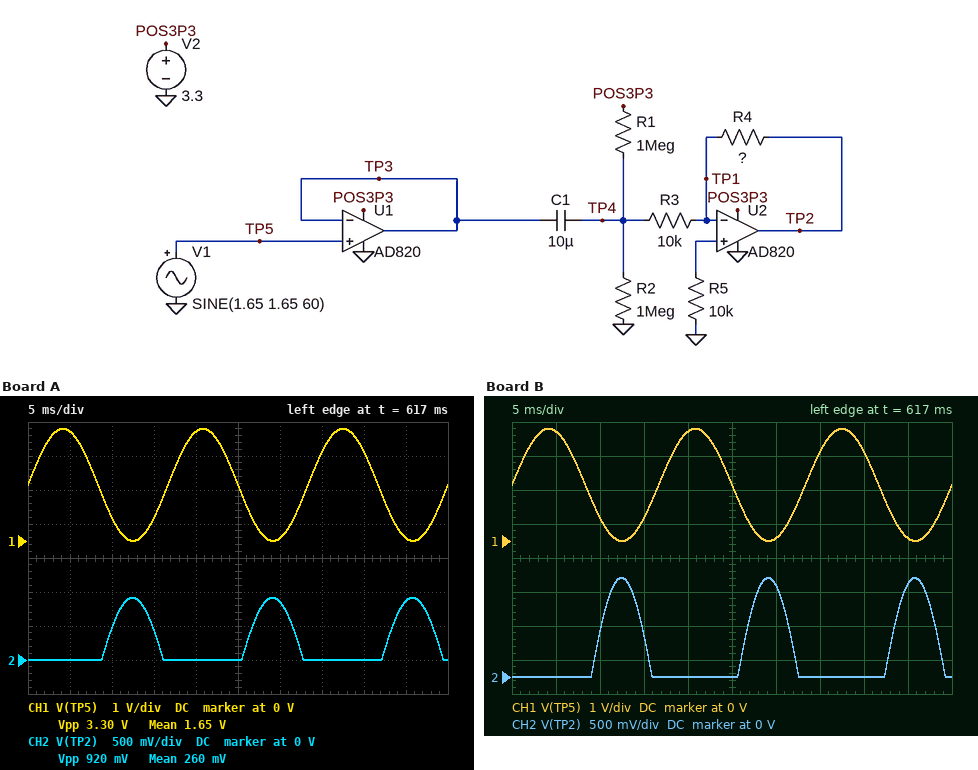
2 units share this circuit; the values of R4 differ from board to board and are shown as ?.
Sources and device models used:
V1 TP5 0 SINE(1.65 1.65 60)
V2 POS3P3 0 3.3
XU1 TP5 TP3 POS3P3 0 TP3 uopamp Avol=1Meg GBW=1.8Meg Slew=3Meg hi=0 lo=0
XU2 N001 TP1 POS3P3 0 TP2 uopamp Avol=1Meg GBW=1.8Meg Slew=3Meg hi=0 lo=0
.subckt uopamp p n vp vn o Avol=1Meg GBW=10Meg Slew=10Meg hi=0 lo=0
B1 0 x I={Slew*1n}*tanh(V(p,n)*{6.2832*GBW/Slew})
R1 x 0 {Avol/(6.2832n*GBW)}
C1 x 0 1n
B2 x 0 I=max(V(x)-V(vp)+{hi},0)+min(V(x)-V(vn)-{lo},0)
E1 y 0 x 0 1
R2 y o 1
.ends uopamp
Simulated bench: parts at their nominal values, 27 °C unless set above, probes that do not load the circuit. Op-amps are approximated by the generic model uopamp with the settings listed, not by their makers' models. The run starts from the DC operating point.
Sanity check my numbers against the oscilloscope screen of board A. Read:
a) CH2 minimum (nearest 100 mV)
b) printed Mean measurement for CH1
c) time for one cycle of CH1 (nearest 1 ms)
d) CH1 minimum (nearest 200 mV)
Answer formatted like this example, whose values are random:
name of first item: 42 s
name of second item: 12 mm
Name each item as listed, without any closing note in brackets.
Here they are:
CH2 minimum: 0 V
printed Mean measurement for CH1: 1.65 V
time for one cycle of CH1: 17 ms
CH1 minimum: 0 V
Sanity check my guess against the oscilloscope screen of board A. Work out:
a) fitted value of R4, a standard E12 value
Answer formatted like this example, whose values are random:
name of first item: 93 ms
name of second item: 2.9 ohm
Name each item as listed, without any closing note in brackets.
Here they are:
fitted value of R4, a standard E12 value: 6.8 kΩ
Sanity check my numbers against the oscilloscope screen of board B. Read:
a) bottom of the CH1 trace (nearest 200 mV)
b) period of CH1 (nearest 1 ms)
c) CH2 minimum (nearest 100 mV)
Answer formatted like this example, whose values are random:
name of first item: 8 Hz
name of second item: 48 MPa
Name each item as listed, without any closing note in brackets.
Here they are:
bottom of the CH1 trace: 0 V
period of CH1: 17 ms
CH2 minimum: 0 V
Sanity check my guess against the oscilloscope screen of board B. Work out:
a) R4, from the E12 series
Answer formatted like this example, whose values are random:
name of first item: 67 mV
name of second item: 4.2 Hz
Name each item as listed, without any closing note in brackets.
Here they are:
R4, from the E12 series: 12 kΩ
